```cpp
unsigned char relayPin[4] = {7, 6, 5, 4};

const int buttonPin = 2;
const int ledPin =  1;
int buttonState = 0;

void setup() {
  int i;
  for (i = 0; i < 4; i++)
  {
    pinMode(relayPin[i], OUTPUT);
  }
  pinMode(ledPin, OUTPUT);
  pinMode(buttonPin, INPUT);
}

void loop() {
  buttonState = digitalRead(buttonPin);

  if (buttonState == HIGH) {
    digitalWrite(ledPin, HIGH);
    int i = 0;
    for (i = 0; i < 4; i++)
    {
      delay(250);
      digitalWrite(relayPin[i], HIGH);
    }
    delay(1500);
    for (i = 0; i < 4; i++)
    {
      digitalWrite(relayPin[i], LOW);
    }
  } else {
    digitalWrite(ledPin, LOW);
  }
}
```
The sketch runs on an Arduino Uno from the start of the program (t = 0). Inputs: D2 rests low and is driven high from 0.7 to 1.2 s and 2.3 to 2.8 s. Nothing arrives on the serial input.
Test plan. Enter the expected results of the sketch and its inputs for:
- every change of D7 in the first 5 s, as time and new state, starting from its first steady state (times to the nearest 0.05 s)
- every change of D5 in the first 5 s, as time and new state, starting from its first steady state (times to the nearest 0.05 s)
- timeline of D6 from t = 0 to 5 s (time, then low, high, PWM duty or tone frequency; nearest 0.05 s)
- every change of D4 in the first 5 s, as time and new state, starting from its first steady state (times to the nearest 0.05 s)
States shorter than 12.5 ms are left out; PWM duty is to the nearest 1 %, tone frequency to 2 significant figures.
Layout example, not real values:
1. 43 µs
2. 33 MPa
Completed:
1. 0 s low; 0.95 s high; 3.2 s low
2. 0 s low; 1.45 s high; 3.2 s low
3. 0 s low; 1.2 s high; 3.2 s low
4. 0 s low; 1.7 s high; 3.2 s low
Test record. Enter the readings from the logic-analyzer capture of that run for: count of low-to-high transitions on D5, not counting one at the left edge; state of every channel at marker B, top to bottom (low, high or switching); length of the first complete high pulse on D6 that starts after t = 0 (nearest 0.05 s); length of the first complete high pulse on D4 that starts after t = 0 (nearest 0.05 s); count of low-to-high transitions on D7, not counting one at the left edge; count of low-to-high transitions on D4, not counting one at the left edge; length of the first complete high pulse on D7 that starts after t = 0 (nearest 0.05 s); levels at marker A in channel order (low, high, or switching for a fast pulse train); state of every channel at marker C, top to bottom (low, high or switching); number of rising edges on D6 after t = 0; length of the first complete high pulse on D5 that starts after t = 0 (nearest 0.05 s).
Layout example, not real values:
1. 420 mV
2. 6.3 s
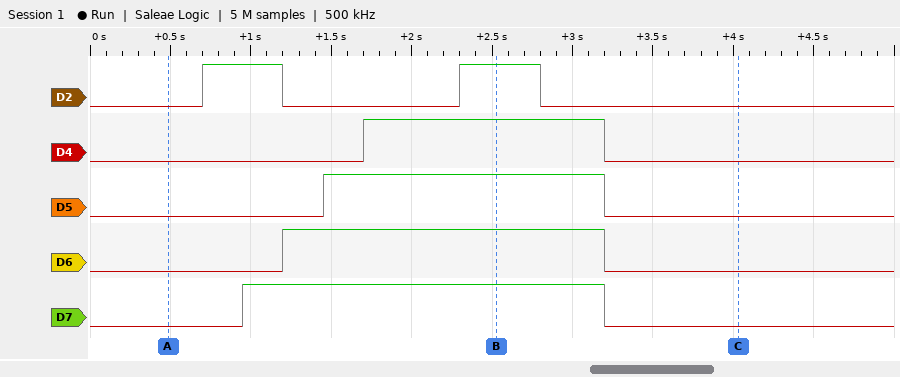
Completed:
1. 1
2. D2 high, D4 high, D5 high, D6 high, D7 high
3. 2.00 s
4. 1.50 s
5. 1
6. 1
7. 2.25 s
8. D2 low, D4 low, D5 low, D6 low, D7 low
9. D2 low, D4 low, D5 low, D6 low, D7 low
10. 1
11. 1.75 s
